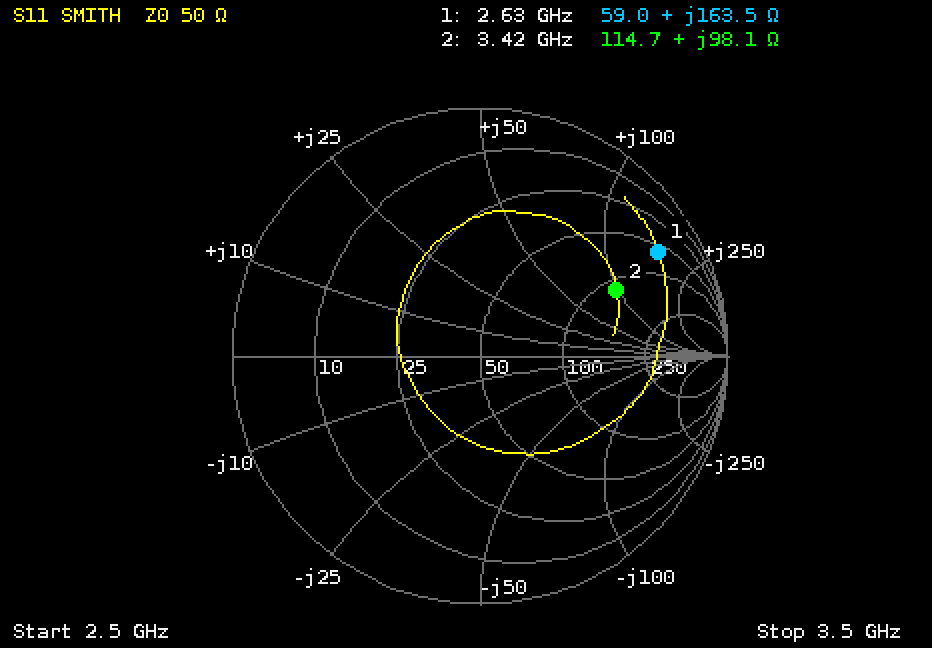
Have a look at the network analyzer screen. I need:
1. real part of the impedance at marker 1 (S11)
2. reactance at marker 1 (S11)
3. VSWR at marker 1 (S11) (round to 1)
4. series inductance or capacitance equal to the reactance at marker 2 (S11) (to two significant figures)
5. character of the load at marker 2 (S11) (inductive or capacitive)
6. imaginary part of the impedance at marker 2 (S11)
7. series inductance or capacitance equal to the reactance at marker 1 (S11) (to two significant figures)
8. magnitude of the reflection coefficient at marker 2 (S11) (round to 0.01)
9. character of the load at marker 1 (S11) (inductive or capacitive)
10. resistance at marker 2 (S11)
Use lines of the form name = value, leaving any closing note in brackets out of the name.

real part of the impedance at marker 1 = 59.0 Ω
reactance at marker 1 = +163.5 Ω
VSWR at marker 1 (S11) = 11
series inductance or capacitance equal to the reactance at marker 2 (S11) = 4.6 nH
character of the load at marker 2 (S11) = inductive
imaginary part of the impedance at marker 2 = +98.1 Ω
series inductance or capacitance equal to the reactance at marker 1 (S11) = 9.9 nH
magnitude of the reflection coefficient at marker 2 (S11) = 0.61
character of the load at marker 1 (S11) = inductive
resistance at marker 2 = 114.7 Ω
